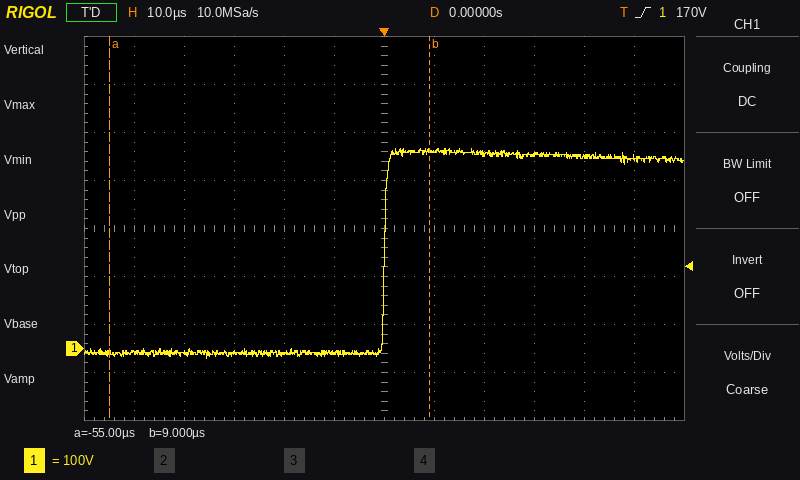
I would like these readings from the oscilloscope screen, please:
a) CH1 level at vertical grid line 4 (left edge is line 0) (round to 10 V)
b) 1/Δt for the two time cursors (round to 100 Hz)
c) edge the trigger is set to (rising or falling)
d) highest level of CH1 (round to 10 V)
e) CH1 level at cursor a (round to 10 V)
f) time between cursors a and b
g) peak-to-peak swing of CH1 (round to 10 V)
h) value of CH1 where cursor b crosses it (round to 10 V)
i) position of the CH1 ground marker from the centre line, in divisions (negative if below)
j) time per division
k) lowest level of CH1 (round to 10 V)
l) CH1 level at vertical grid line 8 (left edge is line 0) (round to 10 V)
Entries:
-10 V
15.6 kHz
rising
420 V
-10 V
64 µs
440 V
410 V
-2.5 div
10 µs
-20 V
410 V
